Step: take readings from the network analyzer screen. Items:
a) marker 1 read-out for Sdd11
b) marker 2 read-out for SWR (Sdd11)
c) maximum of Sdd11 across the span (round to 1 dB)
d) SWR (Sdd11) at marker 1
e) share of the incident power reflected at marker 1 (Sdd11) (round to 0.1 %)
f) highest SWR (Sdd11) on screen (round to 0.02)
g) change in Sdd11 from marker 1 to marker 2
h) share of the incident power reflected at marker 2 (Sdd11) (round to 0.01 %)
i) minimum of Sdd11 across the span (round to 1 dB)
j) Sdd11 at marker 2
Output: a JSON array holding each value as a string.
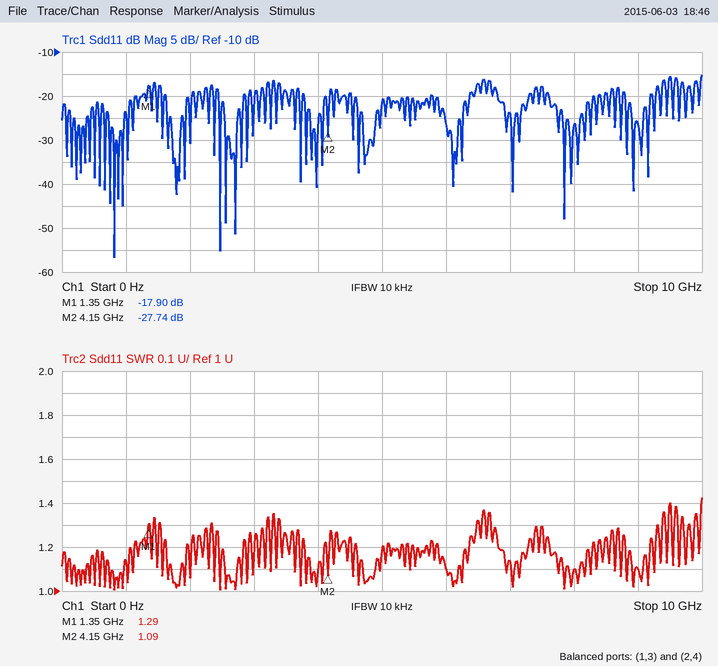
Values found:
["-17.90 dB", "1.09", "-15 dB", "1.29", "1.6 %", "1.42", "-9.84 dB", "0.17 %", "-57 dB", "-27.74 dB"]
